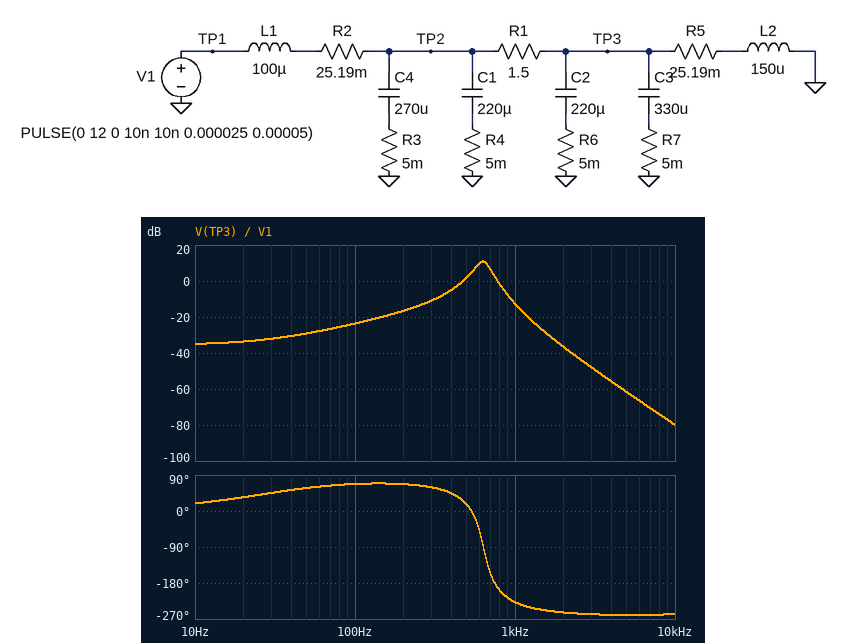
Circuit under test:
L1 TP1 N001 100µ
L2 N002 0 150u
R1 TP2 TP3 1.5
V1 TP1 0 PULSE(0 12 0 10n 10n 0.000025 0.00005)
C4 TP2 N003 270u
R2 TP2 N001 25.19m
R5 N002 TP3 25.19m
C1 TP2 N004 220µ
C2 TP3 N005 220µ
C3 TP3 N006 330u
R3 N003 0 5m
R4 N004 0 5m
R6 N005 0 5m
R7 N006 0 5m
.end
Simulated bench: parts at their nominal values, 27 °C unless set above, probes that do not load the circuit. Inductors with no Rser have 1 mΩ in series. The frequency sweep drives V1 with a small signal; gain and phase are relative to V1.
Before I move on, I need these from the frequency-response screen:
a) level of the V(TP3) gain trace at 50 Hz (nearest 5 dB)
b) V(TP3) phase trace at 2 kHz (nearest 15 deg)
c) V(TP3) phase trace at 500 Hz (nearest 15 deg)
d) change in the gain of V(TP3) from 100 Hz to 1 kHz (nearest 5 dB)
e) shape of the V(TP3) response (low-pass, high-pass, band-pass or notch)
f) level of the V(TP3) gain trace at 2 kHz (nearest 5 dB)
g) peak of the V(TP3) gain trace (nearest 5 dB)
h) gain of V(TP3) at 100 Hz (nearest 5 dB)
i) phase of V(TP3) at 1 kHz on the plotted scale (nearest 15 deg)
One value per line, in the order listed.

-30 dB
-255 deg
15 deg
10 dB
band-pass
-35 dB
10 dB
-25 dB
-225 deg
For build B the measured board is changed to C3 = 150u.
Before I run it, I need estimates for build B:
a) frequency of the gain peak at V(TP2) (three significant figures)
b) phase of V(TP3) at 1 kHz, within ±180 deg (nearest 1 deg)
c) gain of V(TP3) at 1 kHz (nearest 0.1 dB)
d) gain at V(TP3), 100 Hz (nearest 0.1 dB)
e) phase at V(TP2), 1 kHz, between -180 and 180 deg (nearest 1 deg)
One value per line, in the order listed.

700 Hz
141 deg
-8.1 dB
-23.7 dB
-159 deg
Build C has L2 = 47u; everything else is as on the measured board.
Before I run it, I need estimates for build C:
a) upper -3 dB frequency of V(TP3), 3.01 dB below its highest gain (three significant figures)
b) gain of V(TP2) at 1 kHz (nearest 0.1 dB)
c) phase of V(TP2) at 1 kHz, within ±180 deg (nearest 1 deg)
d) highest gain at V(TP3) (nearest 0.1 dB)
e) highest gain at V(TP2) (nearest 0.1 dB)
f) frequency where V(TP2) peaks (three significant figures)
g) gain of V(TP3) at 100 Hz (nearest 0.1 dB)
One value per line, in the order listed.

980 Hz
0.1 dB
-166 deg
0.6 dB
9.8 dB
746 Hz
-31.7 dB
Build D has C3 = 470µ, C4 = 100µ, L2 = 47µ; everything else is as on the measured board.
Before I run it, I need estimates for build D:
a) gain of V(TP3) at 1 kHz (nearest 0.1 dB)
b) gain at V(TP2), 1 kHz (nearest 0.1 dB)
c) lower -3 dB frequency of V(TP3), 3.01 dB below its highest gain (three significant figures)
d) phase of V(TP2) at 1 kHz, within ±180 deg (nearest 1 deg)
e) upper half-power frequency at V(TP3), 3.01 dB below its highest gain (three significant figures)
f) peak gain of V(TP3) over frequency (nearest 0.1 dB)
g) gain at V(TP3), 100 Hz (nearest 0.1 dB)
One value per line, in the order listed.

-0.8 dB
5.7 dB
844 Hz
-139 deg
923 Hz
9.9 dB
-31.7 dB
